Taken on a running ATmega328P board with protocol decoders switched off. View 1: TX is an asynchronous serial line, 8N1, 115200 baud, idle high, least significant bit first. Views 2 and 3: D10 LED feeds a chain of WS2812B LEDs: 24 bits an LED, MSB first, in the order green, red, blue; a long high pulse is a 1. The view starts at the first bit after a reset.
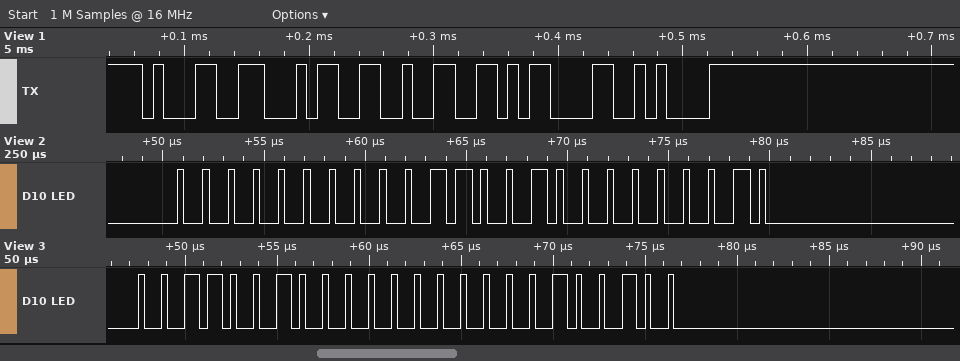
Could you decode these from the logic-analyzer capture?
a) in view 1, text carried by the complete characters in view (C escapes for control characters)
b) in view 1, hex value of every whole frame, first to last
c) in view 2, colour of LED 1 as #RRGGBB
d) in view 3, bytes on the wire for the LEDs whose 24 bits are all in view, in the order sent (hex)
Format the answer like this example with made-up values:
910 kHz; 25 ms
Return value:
"142\r\n"; 31 34 32 0D 0A; #320002; 32 00 24
